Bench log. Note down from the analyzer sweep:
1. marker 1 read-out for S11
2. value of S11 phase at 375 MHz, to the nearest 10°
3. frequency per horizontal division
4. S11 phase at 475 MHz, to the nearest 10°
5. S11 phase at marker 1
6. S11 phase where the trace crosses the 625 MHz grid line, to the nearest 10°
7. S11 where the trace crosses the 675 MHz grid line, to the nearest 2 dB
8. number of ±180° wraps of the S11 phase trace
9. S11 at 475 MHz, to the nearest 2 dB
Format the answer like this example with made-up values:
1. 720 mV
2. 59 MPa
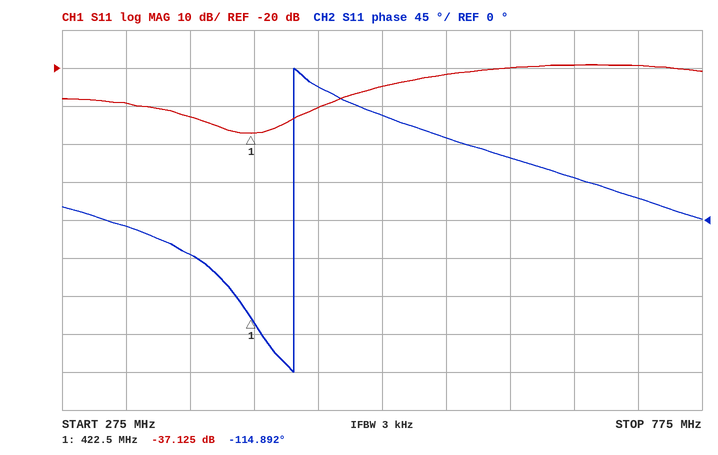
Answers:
1. -37.125 dB
2. -40°
3. 50 MHz
4. 160°
5. -114.892°
6. 70°
7. -20 dB
8. 1
9. -30 dB
